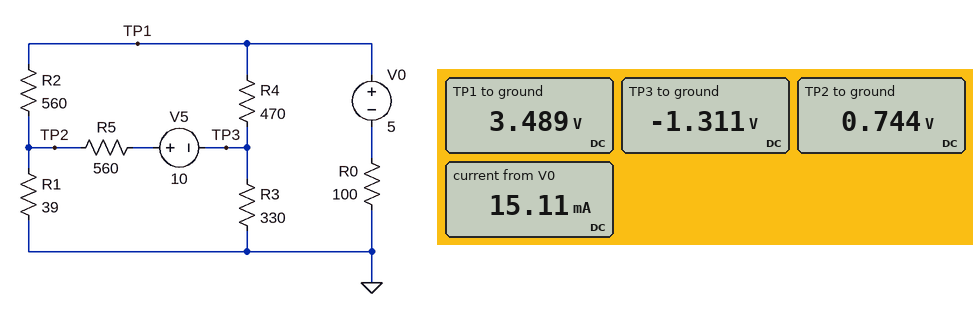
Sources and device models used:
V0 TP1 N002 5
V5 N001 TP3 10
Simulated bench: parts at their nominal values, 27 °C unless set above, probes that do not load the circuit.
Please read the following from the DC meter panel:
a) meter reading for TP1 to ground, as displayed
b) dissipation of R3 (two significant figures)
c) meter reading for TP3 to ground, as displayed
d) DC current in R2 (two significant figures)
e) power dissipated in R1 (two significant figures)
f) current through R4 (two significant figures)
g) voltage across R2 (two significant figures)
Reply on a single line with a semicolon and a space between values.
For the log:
3.489 V; 5.2 mW; -1.311 V; 4.9 mA; 14 mW; 10 mA; 2.7 V
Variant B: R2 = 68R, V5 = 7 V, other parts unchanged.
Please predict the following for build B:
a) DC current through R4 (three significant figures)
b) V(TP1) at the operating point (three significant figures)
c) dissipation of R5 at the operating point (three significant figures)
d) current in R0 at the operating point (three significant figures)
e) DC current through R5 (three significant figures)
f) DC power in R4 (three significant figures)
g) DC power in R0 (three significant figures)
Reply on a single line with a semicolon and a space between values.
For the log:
6.78 mA; 2.41 V; 46.8 mW; 25.9 mA; 9.14 mA; 21.6 mW; 67.3 mW
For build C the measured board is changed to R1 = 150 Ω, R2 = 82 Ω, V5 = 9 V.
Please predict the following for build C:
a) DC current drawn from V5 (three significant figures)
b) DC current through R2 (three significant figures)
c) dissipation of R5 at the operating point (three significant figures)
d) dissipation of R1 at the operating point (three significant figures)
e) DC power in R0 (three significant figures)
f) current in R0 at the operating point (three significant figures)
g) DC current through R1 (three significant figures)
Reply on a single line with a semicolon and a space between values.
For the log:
10.2 mA; 7.93 mA; 58.0 mW; 49.2 mW; 26.7 mW; 16.3 mA; 18.1 mA
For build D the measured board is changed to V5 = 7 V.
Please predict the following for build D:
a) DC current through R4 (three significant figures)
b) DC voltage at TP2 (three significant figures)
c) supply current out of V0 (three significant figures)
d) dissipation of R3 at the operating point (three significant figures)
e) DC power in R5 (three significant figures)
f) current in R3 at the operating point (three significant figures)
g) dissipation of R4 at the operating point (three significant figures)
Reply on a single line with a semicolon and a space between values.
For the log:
8.79 mA; 614 mV; 14.1 mA; 891 µW; 61.0 mW; 1.64 mA; 36.3 mW
